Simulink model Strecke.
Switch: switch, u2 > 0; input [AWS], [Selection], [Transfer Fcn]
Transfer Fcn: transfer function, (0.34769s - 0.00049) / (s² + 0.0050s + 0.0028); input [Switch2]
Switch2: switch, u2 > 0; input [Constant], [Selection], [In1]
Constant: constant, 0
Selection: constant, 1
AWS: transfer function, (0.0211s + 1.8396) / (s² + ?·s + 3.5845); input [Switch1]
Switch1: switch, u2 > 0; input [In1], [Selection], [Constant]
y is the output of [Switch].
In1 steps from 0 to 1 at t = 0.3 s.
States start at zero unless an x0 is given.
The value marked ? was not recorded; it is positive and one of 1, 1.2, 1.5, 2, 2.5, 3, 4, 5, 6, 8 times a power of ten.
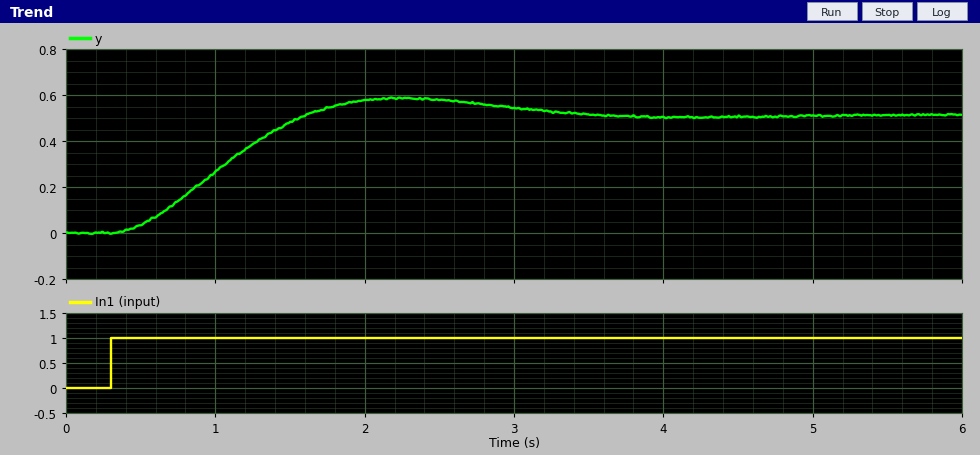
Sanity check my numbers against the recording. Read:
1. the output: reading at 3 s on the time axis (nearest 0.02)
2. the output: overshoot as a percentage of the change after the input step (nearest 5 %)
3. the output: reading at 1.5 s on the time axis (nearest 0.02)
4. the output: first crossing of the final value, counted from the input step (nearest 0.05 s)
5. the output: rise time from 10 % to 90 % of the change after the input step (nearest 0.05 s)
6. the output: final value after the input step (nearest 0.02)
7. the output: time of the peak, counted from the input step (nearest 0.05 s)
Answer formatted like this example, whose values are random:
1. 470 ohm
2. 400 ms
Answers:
1. 0.54
2. 15 %
3. 0.48
4. 1.30 s
5. 0.90 s
6. 0.52
7. 1.95 s
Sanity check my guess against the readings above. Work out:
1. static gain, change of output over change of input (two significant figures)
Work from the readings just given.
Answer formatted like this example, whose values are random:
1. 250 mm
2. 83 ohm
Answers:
1. 0.52
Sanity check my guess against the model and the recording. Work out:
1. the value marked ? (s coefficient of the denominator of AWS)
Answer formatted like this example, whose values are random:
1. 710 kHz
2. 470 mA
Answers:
1. 2
